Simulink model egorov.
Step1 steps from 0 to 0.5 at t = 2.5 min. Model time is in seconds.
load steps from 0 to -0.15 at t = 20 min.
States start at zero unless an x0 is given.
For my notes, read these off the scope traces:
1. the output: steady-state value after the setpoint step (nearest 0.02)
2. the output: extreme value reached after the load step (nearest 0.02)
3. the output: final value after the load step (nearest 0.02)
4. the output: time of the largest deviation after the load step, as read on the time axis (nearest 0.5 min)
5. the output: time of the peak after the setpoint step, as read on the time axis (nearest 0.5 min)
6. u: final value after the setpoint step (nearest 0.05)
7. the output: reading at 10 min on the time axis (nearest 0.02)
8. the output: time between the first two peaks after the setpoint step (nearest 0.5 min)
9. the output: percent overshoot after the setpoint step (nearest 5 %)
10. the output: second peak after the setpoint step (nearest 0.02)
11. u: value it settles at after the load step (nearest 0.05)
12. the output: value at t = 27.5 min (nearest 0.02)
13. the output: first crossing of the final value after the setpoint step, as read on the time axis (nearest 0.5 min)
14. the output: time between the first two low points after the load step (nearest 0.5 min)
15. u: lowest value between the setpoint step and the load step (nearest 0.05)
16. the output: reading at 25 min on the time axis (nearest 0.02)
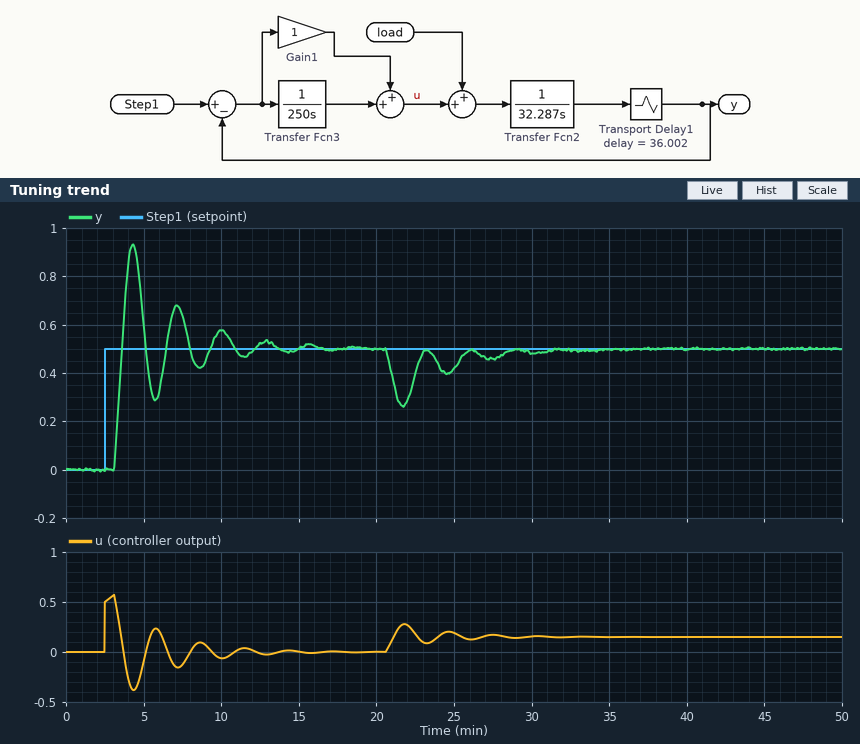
0.50
0.26
0.50
21.5 min
4.5 min
0.00
0.58
3.0 min
85 %
0.68
0.15
0.46
3.5 min
3.0 min
-0.40
0.42
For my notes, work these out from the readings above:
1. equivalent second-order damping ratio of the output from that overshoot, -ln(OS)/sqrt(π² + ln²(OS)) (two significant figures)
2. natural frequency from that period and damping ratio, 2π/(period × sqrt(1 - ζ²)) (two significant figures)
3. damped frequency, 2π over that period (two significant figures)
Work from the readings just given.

0.052
2.1 rad/min
2.1 rad/min
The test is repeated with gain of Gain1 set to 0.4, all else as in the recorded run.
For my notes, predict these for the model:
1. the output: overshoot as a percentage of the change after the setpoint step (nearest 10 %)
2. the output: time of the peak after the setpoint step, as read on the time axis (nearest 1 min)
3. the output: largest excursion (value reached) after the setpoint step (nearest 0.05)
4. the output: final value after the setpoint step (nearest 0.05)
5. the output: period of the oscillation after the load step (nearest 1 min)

60 %
6 min
0.80
0.50
8 min
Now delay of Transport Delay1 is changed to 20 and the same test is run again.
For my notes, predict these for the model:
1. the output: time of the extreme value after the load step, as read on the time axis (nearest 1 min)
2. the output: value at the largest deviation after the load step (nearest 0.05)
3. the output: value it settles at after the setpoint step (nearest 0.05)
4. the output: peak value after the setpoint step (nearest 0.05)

21 min
0.35
0.50
0.65
